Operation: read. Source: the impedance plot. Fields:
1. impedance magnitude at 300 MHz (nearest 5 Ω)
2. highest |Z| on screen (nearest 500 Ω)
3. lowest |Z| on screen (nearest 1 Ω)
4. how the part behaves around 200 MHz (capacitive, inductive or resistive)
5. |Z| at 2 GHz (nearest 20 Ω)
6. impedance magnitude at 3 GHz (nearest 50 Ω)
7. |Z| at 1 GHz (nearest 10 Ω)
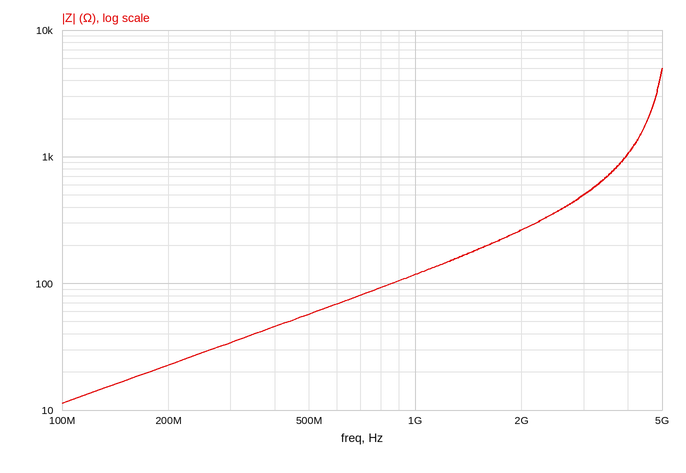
35 Ω
5.0 kΩ
11 Ω
inductive
260 Ω
500 Ω
120 Ω
